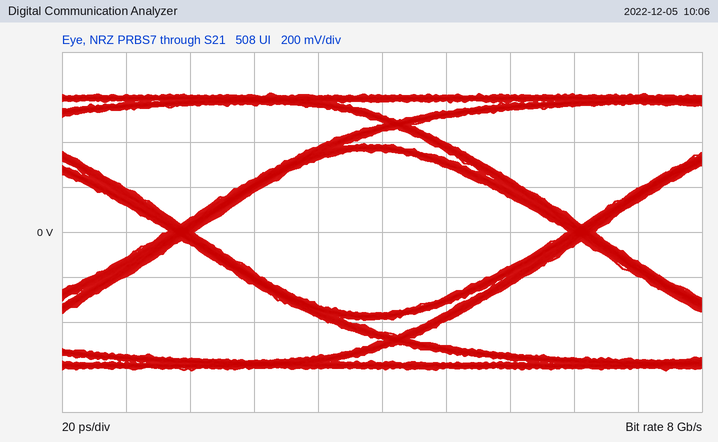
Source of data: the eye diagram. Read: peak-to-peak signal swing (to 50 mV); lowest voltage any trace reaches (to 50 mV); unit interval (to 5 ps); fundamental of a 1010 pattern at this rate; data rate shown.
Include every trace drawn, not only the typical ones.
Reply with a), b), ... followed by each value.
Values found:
a) 1.25 V
b) -600 mV
c) 125 ps
d) 4 GHz
e) 8 Gb/s
